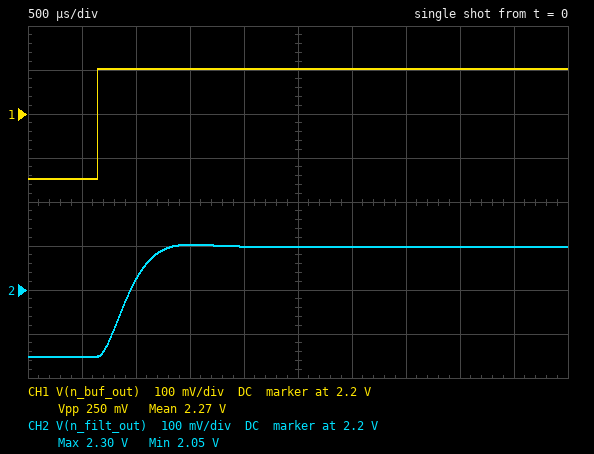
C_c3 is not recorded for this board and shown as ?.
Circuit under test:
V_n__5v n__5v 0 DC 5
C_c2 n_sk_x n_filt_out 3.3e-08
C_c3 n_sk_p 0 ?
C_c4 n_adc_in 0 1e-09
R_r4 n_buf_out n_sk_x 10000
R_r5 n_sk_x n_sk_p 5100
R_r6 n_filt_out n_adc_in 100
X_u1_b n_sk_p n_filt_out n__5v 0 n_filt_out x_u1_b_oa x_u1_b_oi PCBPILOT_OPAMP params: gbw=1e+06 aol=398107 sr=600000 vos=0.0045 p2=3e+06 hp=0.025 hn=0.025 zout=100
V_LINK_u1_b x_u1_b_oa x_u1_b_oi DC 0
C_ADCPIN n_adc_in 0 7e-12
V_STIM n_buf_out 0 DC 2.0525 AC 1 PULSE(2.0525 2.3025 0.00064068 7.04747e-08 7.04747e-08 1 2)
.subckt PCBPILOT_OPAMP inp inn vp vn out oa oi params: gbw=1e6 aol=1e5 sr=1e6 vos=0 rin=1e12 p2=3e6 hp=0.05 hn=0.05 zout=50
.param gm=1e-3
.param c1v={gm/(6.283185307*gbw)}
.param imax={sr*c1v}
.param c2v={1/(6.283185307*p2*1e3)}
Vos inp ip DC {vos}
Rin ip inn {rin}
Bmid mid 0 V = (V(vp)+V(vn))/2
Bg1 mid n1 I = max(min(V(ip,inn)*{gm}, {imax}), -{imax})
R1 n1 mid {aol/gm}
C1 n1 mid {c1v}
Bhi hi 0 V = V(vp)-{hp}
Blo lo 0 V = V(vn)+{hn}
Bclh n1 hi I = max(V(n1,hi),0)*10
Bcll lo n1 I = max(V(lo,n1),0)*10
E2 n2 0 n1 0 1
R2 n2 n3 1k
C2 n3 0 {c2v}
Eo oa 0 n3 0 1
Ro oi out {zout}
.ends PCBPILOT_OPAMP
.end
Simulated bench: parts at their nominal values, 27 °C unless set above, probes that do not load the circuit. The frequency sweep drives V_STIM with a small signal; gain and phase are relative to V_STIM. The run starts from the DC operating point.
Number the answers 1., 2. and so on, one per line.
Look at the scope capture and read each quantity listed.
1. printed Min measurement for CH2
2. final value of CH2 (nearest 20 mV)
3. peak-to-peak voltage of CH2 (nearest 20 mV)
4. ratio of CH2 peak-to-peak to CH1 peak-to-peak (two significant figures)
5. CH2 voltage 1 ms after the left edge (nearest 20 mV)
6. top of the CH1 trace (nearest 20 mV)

1. 2.05 V
2. 2.30 V
3. 260 mV
4. 1.0
5. 2.22 V
6. 2.30 V
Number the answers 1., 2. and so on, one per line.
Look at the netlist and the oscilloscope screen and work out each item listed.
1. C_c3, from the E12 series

1. 18 nF
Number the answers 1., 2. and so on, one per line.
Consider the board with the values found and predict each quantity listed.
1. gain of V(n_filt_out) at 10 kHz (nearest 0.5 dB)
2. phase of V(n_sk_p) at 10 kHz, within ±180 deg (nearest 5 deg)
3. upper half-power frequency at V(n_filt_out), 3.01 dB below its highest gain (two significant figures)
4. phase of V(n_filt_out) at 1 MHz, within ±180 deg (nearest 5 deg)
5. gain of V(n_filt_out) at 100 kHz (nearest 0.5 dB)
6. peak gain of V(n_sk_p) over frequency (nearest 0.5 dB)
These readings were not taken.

1. -41.5 dB
2. -170 deg
3. 820 Hz
4. 25 deg
5. -60.0 dB
6. 0 dB
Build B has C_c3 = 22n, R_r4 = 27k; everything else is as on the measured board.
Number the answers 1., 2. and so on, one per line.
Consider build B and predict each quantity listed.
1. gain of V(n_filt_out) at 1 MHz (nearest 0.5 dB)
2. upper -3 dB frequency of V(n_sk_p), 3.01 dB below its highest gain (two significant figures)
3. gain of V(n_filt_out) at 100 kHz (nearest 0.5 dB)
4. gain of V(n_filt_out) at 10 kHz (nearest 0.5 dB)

1. -49.5 dB
2. 280 Hz
3. -68.5 dB
4. -52.0 dB
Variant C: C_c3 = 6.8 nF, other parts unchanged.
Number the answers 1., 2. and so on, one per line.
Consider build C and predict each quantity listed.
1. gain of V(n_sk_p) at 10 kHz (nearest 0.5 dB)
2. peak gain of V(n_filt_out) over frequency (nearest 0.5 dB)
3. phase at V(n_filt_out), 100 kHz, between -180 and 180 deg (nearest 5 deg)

1. -33.0 dB
2. 1.5 dB
3. 95 deg
